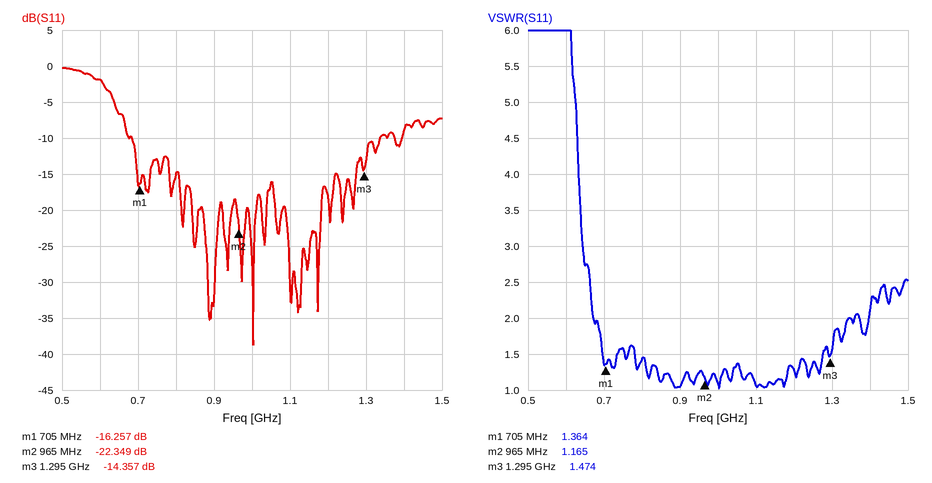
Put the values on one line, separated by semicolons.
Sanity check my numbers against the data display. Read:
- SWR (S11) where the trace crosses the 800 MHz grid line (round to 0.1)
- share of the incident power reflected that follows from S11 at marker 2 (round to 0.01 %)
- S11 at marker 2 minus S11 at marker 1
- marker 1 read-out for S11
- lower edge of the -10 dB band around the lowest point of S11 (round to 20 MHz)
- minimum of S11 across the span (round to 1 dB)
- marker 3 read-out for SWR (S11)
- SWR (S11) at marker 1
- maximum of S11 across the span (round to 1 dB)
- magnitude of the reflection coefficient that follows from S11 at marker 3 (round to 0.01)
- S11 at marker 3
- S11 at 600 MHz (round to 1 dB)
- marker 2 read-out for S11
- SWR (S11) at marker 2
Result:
1.4; 0.58 %; -6.092 dB; -16.257 dB; 680 MHz; -39 dB; 1.474; 1.364; 0 dB; 0.19; -14.357 dB; -2 dB; -22.349 dB; 1.165
